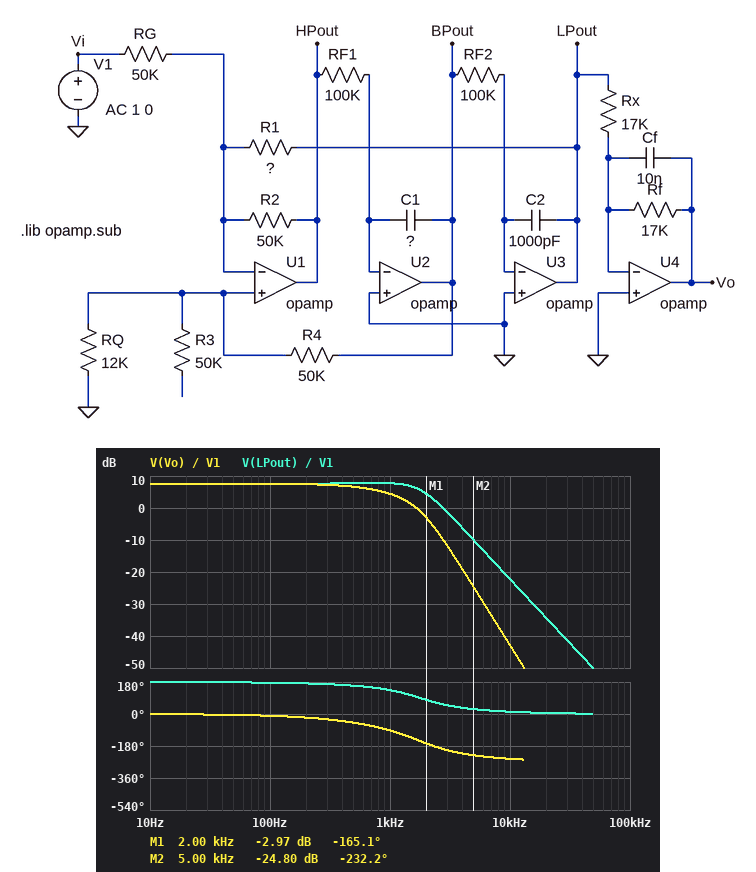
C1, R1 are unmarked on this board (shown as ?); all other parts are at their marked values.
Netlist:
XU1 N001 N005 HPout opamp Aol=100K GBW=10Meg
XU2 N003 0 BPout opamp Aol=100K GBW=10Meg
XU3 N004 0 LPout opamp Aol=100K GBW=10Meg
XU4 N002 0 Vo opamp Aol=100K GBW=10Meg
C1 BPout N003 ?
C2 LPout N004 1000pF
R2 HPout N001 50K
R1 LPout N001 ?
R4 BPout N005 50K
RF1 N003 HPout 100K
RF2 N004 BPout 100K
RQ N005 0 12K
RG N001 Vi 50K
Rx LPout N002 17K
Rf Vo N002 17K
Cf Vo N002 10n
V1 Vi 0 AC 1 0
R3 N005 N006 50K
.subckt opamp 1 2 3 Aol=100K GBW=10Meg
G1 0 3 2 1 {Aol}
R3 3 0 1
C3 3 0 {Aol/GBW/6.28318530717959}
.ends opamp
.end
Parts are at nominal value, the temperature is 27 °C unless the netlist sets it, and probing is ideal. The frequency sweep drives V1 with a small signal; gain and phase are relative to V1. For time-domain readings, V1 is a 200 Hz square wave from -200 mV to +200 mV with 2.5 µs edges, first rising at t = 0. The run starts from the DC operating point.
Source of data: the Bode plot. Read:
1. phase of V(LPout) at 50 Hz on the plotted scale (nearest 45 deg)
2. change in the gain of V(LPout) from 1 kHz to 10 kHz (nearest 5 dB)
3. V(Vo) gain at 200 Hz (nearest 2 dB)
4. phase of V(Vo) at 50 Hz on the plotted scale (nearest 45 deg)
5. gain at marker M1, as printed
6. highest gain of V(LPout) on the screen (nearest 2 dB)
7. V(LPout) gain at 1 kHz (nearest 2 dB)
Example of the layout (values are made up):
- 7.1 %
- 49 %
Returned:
- 180 deg
- -30 dB
- 8 dB
- 0 deg
- -2.97 dB
- 8 dB
- 8 dB
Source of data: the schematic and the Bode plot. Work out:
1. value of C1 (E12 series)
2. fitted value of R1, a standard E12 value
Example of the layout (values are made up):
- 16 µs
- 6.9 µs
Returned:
- 330 pF
- 120 kΩ
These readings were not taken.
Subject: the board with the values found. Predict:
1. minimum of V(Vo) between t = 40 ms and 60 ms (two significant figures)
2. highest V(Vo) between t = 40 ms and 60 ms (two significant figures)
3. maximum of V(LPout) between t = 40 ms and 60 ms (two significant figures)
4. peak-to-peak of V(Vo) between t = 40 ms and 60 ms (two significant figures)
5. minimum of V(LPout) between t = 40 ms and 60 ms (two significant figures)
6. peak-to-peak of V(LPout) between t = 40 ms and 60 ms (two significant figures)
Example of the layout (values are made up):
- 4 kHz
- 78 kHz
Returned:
- -480 mV
- 480 mV
- 560 mV
- 960 mV
- -560 mV
- 1.1 V
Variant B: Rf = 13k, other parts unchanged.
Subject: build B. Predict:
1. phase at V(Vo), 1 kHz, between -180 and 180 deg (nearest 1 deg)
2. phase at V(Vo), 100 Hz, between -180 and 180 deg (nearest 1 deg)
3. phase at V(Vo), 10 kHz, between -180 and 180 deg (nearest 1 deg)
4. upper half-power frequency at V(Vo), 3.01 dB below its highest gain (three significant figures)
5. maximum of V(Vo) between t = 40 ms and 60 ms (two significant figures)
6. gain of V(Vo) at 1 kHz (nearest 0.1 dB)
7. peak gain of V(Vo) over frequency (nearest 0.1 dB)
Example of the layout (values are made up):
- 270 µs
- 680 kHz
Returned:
- -85 deg
- -9 deg
- 110 deg
- 1.20 kHz
- 370 mV
- 3.2 dB
- 5.3 dB
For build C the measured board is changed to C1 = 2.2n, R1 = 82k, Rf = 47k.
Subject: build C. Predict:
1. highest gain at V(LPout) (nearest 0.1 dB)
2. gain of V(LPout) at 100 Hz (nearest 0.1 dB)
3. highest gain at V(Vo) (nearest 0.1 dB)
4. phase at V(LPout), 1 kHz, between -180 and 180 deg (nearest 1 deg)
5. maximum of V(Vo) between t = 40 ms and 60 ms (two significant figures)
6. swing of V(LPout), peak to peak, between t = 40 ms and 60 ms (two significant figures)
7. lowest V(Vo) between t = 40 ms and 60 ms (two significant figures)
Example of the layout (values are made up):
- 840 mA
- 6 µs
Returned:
- 11.7 dB
- 4.4 dB
- 13.1 dB
- 51 deg
- 950 mV
- 1.3 V
- -950 mV
